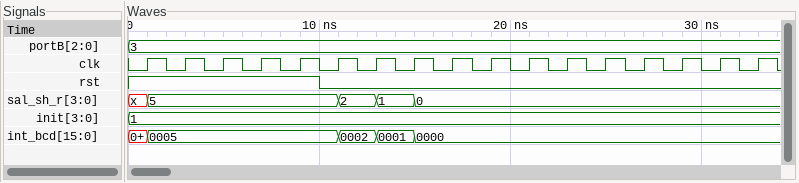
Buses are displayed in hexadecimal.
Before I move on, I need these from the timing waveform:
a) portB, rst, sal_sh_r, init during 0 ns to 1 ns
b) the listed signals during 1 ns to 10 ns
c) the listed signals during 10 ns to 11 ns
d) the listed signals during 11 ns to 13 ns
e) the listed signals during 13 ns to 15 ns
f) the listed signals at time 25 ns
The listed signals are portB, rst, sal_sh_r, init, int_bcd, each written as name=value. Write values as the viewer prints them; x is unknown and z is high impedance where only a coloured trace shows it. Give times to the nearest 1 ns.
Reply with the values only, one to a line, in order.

portB=3, rst=1, sal_sh_r=x, init=1
portB=3, rst=1, sal_sh_r=5, init=1, int_bcd=0005
portB=3, rst=0, sal_sh_r=5, init=1, int_bcd=0005
portB=3, rst=0, sal_sh_r=2, init=1, int_bcd=0002
portB=3, rst=0, sal_sh_r=1, init=1, int_bcd=0001
portB=3, rst=0, sal_sh_r=0, init=1, int_bcd=0000
